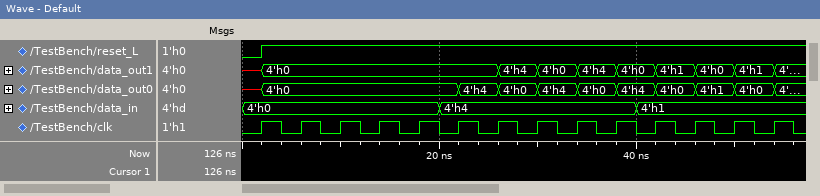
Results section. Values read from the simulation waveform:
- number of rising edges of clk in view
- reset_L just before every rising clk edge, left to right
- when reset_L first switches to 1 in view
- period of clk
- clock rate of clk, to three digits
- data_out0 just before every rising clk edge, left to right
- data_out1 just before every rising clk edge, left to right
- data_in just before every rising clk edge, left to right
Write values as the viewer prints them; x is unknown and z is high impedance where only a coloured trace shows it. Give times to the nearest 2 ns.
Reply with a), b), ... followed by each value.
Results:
a) 14
b) 0 1 1 1 1 1 1 1 1 1 1 1 1 1
c) 2 ns
d) 4 ns
e) 250 MHz
f) x, 4'h0, 4'h0, 4'h0, 4'h0, 4'h0, 4'h4, 4'h0, 4'h4, 4'h0, 4'h4, 4'h0, 4'h1, 4'h0
g) x, 4'h0, 4'h0, 4'h0, 4'h0, 4'h0, 4'h0, 4'h4, 4'h0, 4'h4, 4'h0, 4'h1, 4'h0, 4'h1
h) 4'h0, 4'h0, 4'h0, 4'h0, 4'h0, 4'h4, 4'h4, 4'h4, 4'h4, 4'h4, 4'h1, 4'h1, 4'h1, 4'h1
